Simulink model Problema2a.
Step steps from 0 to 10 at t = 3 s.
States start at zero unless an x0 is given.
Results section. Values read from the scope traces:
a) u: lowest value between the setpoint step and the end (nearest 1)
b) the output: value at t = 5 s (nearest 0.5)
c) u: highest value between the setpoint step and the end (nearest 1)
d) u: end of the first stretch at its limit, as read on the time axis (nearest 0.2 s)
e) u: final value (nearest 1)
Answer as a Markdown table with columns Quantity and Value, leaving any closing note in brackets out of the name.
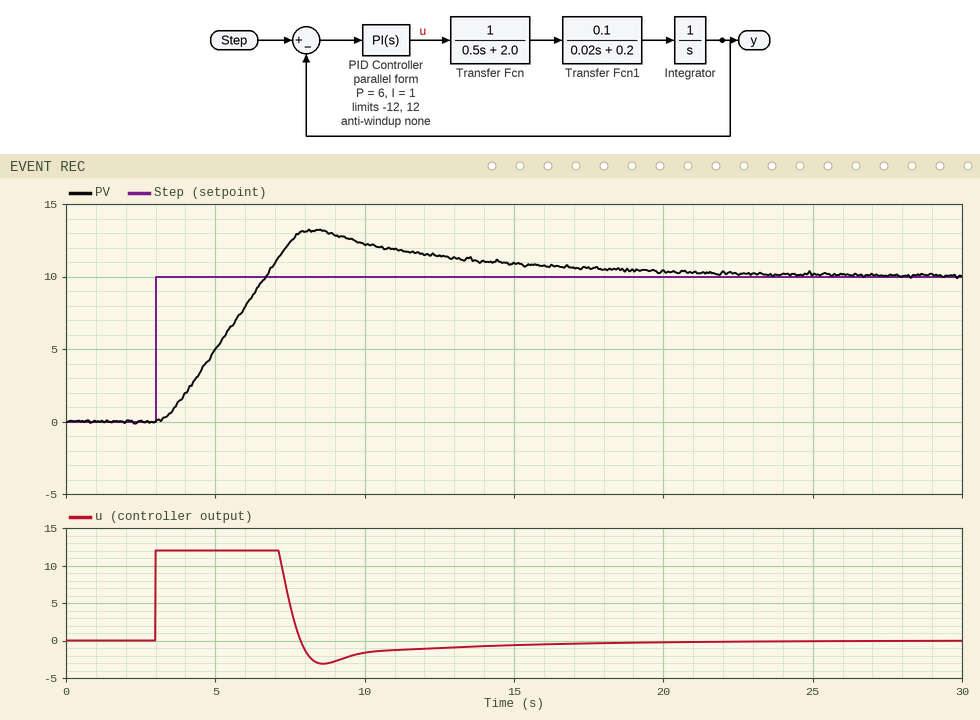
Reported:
| Quantity | Value |
|---|---|
| u: lowest value between the setpoint step and the end | -3 |
| the output: value at t = 5 s | 5.0 |
| u: highest value between the setpoint step and the end | 12 |
| u: end of the first stretch at its limit, as read on the time axis | 7.2 s |
| u: final value | 0 |
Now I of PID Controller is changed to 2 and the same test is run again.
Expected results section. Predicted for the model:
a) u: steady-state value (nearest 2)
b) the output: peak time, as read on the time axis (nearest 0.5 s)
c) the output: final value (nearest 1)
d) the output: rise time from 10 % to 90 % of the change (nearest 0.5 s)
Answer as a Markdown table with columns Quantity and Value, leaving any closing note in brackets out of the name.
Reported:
| Quantity | Value |
|---|---|
| u: steady-state value | 0 |
| the output: peak time, as read on the time axis | 9.0 s |
| the output: final value | 10 |
| the output: rise time from 10 % to 90 % of the change | 2.5 s |
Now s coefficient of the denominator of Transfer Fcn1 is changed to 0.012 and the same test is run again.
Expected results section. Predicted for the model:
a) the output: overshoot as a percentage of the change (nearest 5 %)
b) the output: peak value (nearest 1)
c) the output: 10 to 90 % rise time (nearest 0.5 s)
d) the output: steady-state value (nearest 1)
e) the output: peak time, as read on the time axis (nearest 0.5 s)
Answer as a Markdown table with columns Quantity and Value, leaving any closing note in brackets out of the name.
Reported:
| Quantity | Value |
|---|---|
| the output: overshoot as a percentage of the change | 30 % |
| the output: peak value | 13 |
| the output: 10 to 90 % rise time | 2.5 s |
| the output: steady-state value | 10 |
| the output: peak time, as read on the time axis | 8.0 s |
